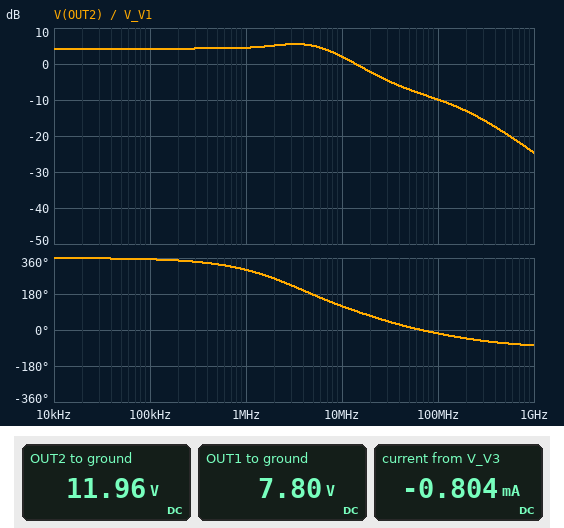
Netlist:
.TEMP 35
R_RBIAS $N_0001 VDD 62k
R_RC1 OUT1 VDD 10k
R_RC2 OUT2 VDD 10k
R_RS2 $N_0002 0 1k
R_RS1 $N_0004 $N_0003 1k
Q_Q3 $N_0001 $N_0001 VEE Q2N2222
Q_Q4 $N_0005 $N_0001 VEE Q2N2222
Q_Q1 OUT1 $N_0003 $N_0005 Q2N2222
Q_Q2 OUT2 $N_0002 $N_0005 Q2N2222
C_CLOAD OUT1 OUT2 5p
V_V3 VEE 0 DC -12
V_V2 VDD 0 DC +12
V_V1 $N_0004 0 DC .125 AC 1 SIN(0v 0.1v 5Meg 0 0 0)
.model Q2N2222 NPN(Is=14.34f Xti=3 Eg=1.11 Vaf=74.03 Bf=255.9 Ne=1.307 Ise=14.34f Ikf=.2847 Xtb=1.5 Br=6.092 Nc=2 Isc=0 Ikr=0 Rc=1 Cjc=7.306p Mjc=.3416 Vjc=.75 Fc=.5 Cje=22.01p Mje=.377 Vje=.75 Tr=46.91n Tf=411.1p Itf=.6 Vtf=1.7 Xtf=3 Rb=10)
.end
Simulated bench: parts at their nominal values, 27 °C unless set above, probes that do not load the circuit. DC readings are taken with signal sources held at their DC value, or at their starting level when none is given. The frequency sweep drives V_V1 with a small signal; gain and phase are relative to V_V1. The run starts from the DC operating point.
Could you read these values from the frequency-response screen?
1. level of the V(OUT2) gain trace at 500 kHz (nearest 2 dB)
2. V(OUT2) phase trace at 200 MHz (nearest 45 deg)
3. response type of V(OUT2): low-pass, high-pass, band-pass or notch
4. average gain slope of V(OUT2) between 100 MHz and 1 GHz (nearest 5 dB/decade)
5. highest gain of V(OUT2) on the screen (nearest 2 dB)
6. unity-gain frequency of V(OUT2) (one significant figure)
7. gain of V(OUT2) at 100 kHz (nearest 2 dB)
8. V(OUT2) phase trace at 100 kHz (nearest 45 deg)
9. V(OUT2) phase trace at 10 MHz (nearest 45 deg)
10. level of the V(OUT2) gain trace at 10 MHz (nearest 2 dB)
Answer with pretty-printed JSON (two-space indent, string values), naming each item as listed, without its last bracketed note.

{
  "level of the V(OUT2) gain trace at 500 kHz": "4 dB",
  "V(OUT2) phase trace at 200 MHz": "-45 deg",
  "response type of V(OUT2): low-pass, high-pass, band-pass or notch": "low-pass",
  "average gain slope of V(OUT2) between 100 MHz and 1 GHz": "-15 dB/decade",
  "highest gain of V(OUT2) on the screen": "6 dB",
  "unity-gain frequency of V(OUT2)": "10 MHz",
  "gain of V(OUT2) at 100 kHz": "4 dB",
  "V(OUT2) phase trace at 100 kHz": "360 deg",
  "V(OUT2) phase trace at 10 MHz": "135 deg",
  "level of the V(OUT2) gain trace at 10 MHz": "2 dB"
}
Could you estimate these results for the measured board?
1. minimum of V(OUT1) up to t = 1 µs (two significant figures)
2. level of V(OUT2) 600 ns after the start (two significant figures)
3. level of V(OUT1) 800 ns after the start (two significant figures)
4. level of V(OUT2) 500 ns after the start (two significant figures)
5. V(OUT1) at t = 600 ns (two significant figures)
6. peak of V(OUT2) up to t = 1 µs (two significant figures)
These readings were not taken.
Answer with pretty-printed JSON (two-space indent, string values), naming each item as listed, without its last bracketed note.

{
  "minimum of V(OUT1) up to t = 1 µs": "9.4 V",
  "level of V(OUT2) 600 ns after the start": "9.7 V",
  "level of V(OUT1) 800 ns after the start": "10 V",
  "level of V(OUT2) 500 ns after the start": "10 V",
  "V(OUT1) at t = 600 ns": "10 V",
  "peak of V(OUT2) up to t = 1 µs": "10 V"
}
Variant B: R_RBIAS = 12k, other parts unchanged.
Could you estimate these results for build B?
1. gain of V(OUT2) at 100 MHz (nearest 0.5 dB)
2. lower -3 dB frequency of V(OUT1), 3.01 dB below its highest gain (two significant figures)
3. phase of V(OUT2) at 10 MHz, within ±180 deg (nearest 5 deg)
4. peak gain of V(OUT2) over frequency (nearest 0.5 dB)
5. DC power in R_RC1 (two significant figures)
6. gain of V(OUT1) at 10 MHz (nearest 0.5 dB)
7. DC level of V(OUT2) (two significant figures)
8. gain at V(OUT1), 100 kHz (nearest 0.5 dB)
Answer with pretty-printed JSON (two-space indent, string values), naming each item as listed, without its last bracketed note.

{
  "gain of V(OUT2) at 100 MHz": "-15.5 dB",
  "lower -3 dB frequency of V(OUT1), 3.01 dB below its highest gain": "1.4 MHz",
  "phase of V(OUT2) at 10 MHz, within ±180 deg": "-90 deg",
  "peak gain of V(OUT2) over frequency": "19.0 dB",
  "DC power in R_RC1": "16 mW",
  "gain of V(OUT1) at 10 MHz": "-6.5 dB",
  "DC level of V(OUT2)": "3.7 V",
  "gain at V(OUT1), 100 kHz": "-18.0 dB"
}
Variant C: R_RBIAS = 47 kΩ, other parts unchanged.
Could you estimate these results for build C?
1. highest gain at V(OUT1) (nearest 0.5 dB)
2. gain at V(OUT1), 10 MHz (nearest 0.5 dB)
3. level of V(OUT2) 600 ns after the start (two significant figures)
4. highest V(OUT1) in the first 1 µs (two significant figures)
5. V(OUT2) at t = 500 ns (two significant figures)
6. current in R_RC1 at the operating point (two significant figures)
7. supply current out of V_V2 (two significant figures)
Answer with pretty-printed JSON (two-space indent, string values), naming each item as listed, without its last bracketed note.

{
  "highest gain at V(OUT1)": "9.0 dB",
  "gain at V(OUT1), 10 MHz": "6.0 dB",
  "level of V(OUT2) 600 ns after the start": "9.0 V",
  "highest V(OUT1) in the first 1 µs": "9.5 V",
  "V(OUT2) at t = 500 ns": "9.6 V",
  "current in R_RC1 at the operating point": "550 µA",
  "supply current out of V_V2": "1.1 mA"
}
